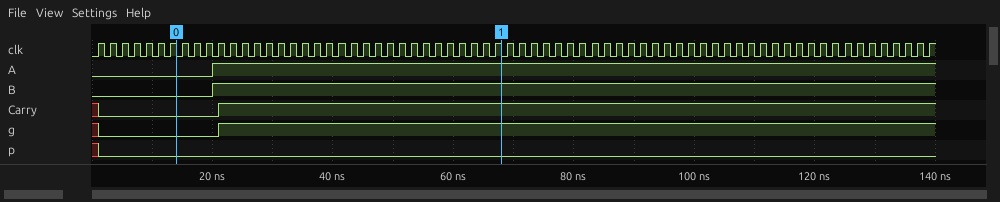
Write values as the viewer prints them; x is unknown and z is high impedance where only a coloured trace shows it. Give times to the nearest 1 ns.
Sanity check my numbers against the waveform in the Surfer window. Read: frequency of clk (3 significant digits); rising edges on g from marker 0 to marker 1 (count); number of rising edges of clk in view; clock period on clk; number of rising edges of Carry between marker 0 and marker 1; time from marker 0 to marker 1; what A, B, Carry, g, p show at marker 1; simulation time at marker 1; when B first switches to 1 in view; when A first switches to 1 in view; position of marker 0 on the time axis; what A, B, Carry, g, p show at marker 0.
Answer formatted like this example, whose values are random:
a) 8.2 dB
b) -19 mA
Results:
a) 500 MHz
b) 1
c) 70
d) 2 ns
e) 1
f) 54 ns
g) A=1, B=1, Carry=1, g=1, p=0
h) 68 ns
i) 20 ns
j) 20 ns
k) 14 ns
l) A=0, B=0, Carry=0, g=0, p=0
